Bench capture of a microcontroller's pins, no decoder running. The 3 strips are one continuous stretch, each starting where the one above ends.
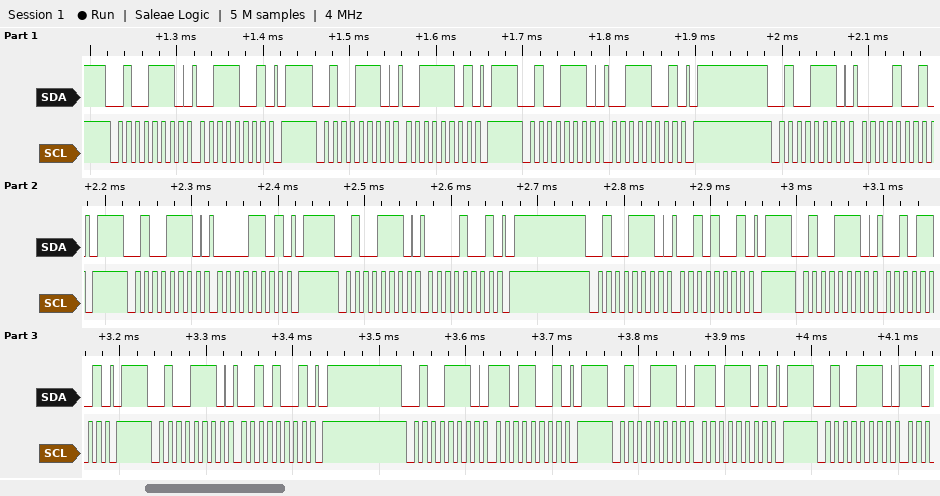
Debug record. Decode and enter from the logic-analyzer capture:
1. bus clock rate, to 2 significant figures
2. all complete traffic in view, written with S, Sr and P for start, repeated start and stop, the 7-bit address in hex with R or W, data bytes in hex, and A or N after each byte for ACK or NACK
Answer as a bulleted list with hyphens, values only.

- 100 kHz
- S 27W A 39 A P S 27W A 3D A P S 27W A 39 A P S 27W A 09 A P S 27W A 0D A P S 27W A 09 A P S 27W A 29 A P S 27W A 2D A P S 27W A 29 A P S 27W A D9 A P S 27W A DD A P S 27W A
